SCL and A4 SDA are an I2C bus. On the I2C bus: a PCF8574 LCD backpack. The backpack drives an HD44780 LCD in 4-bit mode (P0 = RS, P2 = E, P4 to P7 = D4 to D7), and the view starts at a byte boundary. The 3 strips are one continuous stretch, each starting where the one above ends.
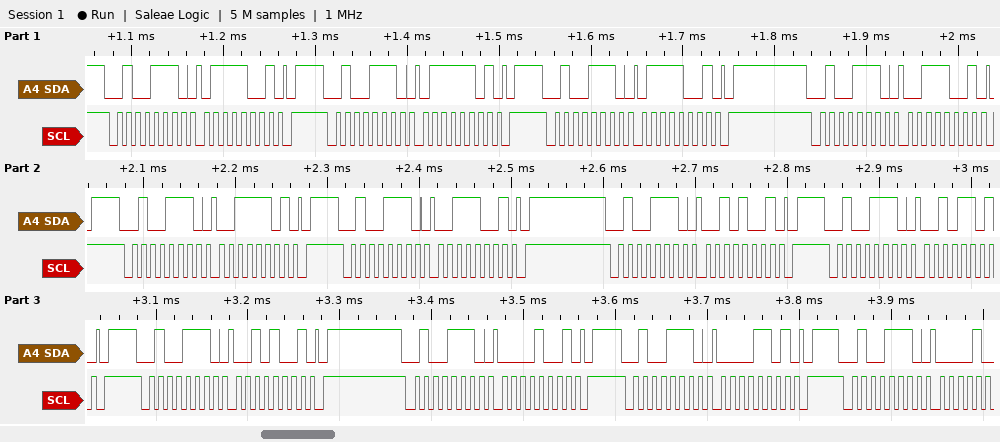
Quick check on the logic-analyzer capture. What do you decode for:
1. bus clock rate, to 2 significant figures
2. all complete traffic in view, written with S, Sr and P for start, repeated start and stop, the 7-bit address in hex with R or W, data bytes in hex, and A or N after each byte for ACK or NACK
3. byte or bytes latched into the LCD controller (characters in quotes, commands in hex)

100 kHz
S 27W A 79 A P S 27W A 7D A P S 27W A 79 A P S 27W A 39 A P S 27W A 3D A P S 27W A 39 A P S 27W A 29 A P S 27W A 2D A P S 27W A 29 A P S 27W A 09 A P S 27W A 0D A P S 27W A
's'
